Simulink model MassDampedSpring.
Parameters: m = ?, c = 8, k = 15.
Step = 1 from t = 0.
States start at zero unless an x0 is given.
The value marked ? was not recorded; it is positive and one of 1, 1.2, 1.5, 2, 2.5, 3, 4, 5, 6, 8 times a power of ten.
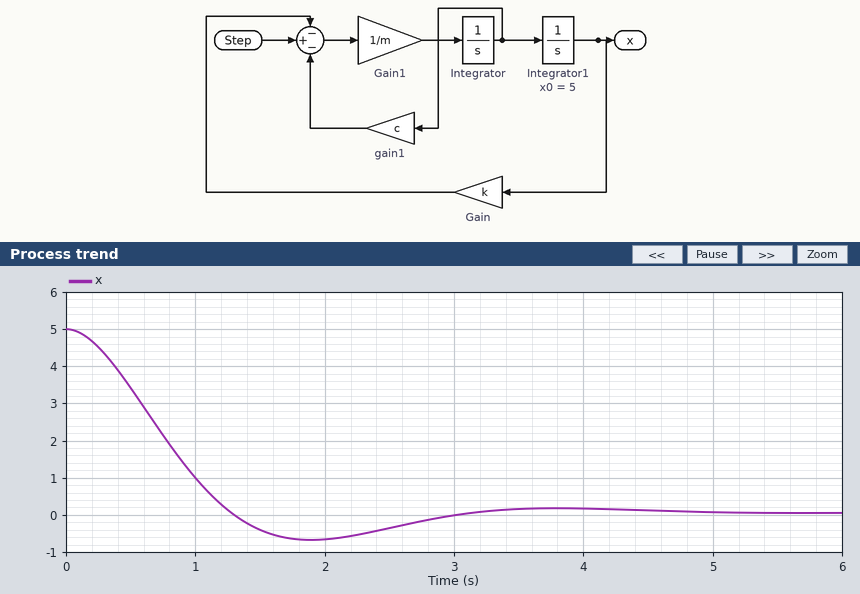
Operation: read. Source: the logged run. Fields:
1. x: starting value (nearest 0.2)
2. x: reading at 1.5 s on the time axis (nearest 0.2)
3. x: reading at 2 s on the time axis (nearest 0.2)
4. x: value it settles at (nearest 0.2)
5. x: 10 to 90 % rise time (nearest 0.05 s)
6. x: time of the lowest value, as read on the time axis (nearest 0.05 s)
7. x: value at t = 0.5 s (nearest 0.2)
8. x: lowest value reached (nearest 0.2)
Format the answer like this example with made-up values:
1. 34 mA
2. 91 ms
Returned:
1. 5.0
2. -0.4
3. -0.6
4. 0.0
5. 0.85 s
6. 1.90 s
7. 3.4
8. -0.6
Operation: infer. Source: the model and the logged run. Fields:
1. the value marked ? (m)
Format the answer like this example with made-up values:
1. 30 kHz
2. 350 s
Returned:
1. 4
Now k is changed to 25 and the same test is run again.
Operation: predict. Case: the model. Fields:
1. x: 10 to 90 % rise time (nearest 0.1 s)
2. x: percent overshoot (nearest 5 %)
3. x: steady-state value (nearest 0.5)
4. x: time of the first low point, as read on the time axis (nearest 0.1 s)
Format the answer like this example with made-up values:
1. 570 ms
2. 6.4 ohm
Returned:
1. 0.6 s
2. 25 %
3. 0.0
4. 1.4 s
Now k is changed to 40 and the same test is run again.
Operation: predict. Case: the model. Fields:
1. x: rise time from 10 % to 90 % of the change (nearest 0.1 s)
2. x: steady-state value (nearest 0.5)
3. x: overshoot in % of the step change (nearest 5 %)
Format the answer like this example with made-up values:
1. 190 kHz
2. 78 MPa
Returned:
1. 0.4 s
2. 0.0
3. 35 %
